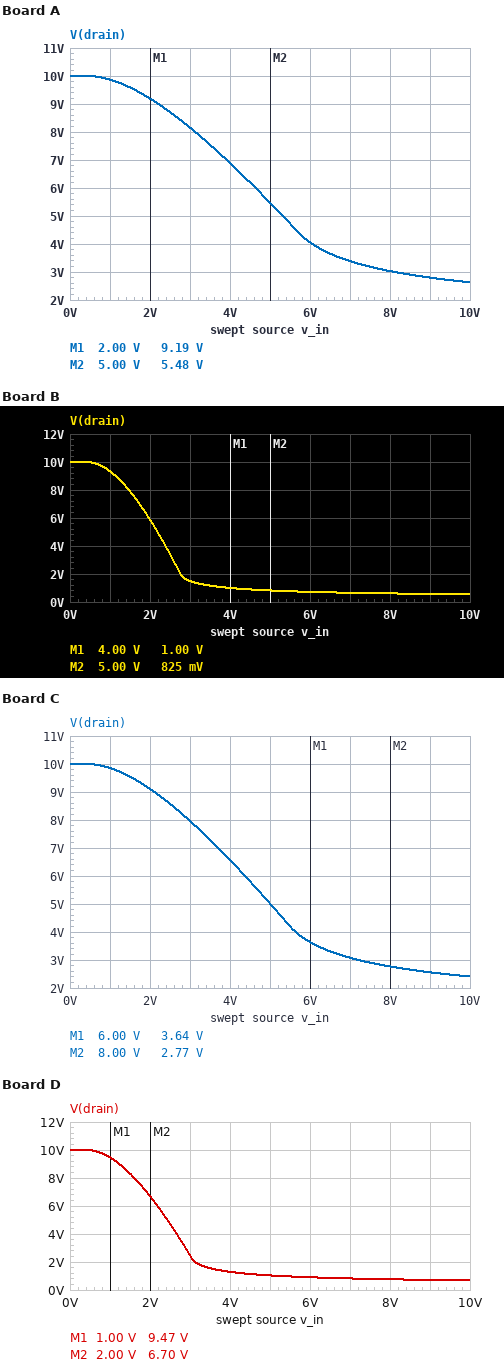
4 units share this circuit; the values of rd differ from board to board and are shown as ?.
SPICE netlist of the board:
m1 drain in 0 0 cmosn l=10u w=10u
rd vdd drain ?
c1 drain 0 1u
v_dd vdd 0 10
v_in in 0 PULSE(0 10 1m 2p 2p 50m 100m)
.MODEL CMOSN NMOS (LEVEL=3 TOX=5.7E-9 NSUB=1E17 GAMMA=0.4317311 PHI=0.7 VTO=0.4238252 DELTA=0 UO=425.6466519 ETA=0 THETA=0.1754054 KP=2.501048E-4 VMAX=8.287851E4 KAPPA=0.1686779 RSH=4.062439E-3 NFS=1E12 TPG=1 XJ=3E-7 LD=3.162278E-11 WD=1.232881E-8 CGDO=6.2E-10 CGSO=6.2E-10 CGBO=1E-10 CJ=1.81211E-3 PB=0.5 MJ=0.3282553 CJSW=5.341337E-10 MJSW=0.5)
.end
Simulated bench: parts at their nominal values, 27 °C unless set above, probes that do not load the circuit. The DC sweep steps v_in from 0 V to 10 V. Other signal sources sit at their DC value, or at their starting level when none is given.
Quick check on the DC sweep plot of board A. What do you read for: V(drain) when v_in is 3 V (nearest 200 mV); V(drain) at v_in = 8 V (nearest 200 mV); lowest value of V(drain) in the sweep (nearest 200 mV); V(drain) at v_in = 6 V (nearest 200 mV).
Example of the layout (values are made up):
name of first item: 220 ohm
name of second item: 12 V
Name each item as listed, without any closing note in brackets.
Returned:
V(drain) when v_in is 3 V: 8.2 V
V(drain) at v_in = 8 V: 3.0 V
lowest value of V(drain) in the sweep: 2.6 V
V(drain) at v_in = 6 V: 4.0 V
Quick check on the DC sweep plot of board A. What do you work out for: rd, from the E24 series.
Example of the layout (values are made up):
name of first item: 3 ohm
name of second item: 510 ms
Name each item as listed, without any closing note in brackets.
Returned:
rd, from the E24 series: 3.9 kΩ
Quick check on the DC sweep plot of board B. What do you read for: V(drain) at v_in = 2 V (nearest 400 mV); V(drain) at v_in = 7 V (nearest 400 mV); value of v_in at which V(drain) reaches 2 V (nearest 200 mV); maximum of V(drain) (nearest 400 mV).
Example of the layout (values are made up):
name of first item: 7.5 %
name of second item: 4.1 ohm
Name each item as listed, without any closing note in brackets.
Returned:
V(drain) at v_in = 2 V: 6.0 V
V(drain) at v_in = 7 V: 800 mV
value of v_in at which V(drain) reaches 2 V: 2.8 V
maximum of V(drain): 10.0 V
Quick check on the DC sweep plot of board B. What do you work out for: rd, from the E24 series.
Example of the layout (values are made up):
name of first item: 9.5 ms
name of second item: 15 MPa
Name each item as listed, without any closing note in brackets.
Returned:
rd, from the E24 series: 20 kΩ
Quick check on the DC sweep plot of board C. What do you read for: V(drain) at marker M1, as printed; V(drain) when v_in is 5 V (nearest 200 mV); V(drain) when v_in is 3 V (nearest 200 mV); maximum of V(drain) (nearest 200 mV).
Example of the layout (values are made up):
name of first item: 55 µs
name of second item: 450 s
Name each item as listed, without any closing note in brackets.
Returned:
V(drain) at marker M1, as printed: 3.64 V
V(drain) when v_in is 5 V: 5.0 V
V(drain) when v_in is 3 V: 8.0 V
maximum of V(drain): 10.0 V
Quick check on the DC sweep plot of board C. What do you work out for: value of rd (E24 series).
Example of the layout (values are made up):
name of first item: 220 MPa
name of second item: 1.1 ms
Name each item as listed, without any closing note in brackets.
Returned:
value of rd: 4.3 kΩ
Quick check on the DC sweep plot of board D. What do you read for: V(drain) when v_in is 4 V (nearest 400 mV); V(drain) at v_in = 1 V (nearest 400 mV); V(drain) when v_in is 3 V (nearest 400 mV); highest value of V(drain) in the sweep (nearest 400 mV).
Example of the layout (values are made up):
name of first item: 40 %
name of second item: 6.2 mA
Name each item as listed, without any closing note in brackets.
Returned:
V(drain) when v_in is 4 V: 1.2 V
V(drain) at v_in = 1 V: 9.6 V
V(drain) when v_in is 3 V: 2.4 V
highest value of V(drain) in the sweep: 10.0 V
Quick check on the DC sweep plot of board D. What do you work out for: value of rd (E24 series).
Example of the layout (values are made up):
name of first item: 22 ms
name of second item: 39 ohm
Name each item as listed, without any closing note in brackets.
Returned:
value of rd: 16 kΩ
